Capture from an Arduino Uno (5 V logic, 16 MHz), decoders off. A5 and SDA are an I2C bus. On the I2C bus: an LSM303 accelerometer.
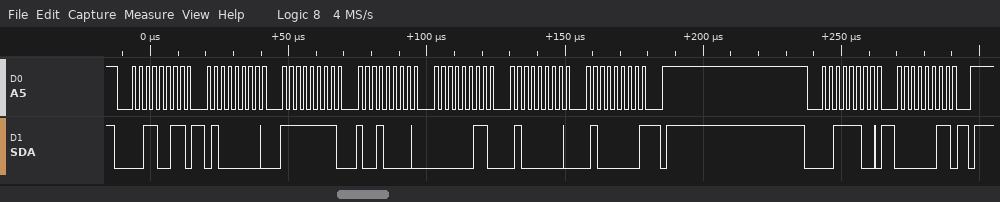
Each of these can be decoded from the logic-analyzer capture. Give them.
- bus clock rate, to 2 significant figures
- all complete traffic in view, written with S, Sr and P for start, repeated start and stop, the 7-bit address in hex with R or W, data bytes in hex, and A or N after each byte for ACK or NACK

400 kHz
S 19R A 40 A FF A 90 A 03 A 40 A 40 N P S 1EW A 03 A P
